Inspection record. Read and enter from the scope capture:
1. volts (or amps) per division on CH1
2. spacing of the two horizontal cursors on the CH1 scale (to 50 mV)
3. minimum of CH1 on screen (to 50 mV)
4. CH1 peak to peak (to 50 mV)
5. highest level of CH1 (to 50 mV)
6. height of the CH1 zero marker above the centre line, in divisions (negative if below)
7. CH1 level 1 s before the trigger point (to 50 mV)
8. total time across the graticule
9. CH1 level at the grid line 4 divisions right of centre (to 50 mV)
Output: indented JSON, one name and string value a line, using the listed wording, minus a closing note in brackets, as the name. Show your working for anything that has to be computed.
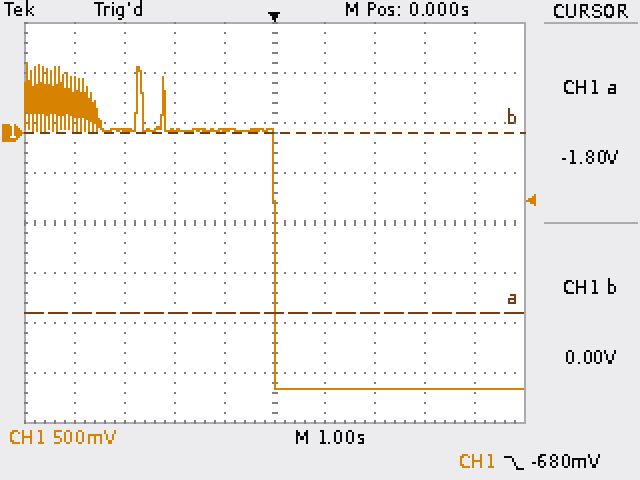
{
  "volts (or amps) per division on CH1": "500 mV",
  "spacing of the two horizontal cursors on the CH1 scale": "1.80 V",
  "minimum of CH1 on screen": "-2.55 V",
  "CH1 peak to peak": "700 mV − (-2.55 V) = 3.25 V",
  "highest level of CH1": "700 mV",
  "height of the CH1 zero marker above the centre line, in divisions": "+1.8 div",
  "CH1 level 1 s before the trigger point": "50 mV",
  "total time across the graticule": "10 s",
  "CH1 level at the grid line 4 divisions right of centre": "-2.55 V"
}
